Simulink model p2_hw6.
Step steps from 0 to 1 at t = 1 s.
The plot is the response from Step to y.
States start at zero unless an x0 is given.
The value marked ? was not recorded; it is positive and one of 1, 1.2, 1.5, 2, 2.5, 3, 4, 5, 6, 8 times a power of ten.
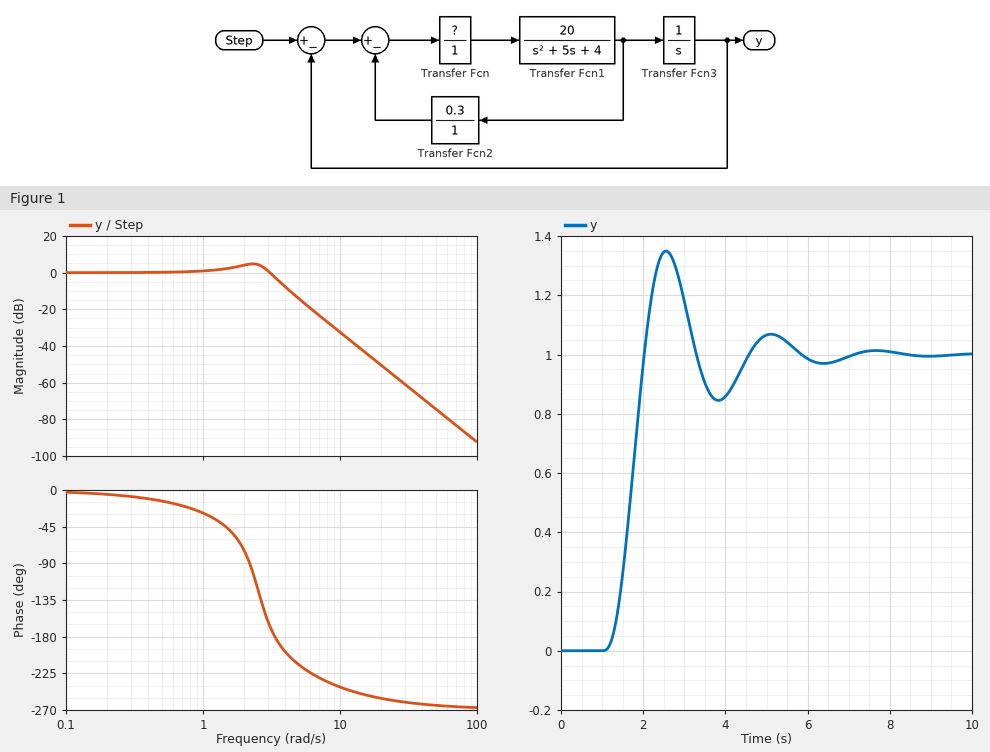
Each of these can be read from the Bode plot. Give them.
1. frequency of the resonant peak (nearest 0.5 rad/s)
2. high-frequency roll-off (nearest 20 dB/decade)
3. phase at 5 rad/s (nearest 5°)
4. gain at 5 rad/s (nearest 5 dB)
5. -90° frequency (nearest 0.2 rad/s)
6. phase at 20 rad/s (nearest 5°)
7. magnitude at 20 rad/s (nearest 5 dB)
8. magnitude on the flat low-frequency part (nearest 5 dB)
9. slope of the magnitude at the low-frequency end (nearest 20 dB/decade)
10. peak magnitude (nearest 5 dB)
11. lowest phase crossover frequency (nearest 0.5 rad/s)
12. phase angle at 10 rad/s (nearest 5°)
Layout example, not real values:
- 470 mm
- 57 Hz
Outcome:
- 2.5 rad/s
- -60 dB/decade
- -215°
- -15 dB
- 2.2 rad/s
- -255°
- -50 dB
- 0 dB
- 0 dB/decade
- 5 dB
- 3.5 rad/s
- -240°
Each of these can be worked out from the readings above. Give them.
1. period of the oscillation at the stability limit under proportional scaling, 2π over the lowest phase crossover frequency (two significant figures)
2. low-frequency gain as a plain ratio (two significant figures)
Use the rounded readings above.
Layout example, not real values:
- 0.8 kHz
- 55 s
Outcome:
- 1.8 s
- 1.0
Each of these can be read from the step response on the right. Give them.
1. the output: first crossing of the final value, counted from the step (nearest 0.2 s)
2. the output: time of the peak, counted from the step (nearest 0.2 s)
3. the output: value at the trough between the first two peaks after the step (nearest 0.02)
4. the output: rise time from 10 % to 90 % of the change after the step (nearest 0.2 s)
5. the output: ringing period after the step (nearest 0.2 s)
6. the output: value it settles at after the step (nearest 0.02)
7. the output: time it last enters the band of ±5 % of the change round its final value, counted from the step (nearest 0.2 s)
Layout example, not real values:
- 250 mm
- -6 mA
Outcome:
- 1.0 s
- 1.6 s
- 0.84
- 0.6 s
- 2.6 s
- 1.00
- 4.4 s
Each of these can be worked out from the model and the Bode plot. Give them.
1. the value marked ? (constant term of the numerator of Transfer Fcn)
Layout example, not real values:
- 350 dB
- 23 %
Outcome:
- 1.2
